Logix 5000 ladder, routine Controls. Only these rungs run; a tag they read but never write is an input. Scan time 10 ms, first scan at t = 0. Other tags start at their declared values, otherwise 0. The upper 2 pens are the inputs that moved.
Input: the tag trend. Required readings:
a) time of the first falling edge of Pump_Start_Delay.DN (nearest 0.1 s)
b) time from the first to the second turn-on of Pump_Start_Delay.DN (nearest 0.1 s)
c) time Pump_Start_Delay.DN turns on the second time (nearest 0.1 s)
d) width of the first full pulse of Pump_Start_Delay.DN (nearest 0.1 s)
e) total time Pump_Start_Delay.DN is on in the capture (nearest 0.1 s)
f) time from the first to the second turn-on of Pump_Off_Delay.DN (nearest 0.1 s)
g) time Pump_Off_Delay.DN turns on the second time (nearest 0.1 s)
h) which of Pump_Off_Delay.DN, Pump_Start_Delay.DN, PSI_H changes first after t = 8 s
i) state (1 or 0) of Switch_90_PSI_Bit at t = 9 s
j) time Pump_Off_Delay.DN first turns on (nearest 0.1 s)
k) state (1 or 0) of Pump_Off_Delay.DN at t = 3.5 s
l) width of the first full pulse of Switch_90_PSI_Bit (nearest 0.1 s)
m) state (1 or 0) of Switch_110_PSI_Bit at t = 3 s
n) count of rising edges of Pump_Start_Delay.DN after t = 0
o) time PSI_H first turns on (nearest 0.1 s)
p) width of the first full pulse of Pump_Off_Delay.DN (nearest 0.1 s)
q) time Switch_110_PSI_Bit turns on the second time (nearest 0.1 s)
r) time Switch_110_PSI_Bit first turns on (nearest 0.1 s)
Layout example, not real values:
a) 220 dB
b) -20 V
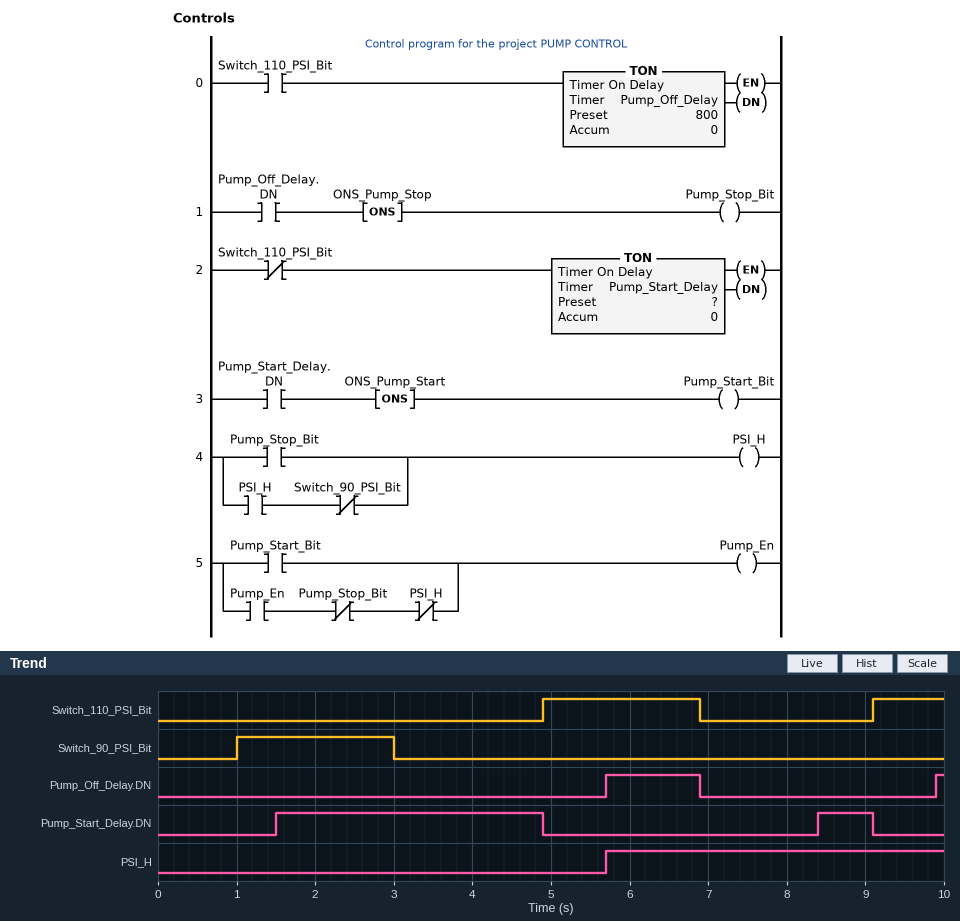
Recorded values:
a) 4.9 s
b) 6.9 s
c) 8.4 s
d) 3.4 s
e) 4.1 s
f) 4.2 s
g) 9.9 s
h) Pump_Start_Delay.DN
i) 0
j) 5.7 s
k) 0
l) 2.0 s
m) 0
n) 2
o) 5.7 s
p) 1.2 s
q) 9.1 s
r) 4.9 s
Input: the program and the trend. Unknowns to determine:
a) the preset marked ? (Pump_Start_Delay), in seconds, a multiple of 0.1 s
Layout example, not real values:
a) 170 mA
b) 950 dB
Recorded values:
a) 1.5 s
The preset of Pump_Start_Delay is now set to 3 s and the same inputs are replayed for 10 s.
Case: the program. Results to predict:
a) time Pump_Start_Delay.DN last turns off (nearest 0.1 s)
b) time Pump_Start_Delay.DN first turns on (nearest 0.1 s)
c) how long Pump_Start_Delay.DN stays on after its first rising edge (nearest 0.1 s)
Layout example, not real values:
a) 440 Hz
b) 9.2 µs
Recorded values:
a) 4.9 s
b) 3.0 s
c) 1.9 s
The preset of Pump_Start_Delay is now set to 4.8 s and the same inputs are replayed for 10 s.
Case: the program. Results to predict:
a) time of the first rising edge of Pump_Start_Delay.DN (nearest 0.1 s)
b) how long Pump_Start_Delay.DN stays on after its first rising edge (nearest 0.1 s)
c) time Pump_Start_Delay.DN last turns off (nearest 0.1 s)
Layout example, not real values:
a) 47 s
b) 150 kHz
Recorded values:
a) 4.8 s
b) 0.1 s
c) 4.9 s
